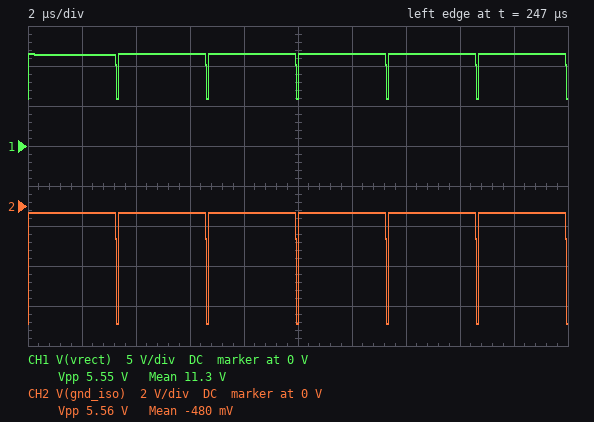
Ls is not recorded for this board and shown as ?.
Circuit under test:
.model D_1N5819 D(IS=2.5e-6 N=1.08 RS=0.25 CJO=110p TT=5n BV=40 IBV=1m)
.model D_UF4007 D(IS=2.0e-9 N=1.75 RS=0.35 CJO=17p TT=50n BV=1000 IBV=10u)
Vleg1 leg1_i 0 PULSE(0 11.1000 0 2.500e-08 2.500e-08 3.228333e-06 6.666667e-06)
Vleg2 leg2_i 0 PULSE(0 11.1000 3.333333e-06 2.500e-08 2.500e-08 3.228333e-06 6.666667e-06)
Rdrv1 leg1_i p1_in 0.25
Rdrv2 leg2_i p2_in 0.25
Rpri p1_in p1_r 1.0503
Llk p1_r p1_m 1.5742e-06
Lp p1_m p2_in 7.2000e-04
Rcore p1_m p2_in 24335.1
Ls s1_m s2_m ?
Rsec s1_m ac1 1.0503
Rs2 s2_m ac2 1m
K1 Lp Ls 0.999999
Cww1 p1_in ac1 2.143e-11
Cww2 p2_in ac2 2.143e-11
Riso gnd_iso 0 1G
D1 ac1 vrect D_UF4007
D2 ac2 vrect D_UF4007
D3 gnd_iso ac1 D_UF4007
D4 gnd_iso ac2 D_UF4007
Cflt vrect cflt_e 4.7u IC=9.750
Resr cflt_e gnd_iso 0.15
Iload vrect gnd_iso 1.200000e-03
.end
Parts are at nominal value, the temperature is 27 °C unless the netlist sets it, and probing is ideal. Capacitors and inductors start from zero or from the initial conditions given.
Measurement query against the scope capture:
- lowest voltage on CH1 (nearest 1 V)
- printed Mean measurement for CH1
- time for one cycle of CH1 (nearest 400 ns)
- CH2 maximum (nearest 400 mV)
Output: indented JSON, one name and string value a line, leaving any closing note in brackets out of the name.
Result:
{
  "lowest voltage on CH1": "6 V",
  "printed Mean measurement for CH1": "11.3 V",
  "time for one cycle of CH1": "3.2 µs",
  "CH2 maximum": "-400 mV"
}
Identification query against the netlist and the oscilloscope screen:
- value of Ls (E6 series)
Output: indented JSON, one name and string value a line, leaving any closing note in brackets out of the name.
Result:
{
  "value of Ls": "1 mH"
}
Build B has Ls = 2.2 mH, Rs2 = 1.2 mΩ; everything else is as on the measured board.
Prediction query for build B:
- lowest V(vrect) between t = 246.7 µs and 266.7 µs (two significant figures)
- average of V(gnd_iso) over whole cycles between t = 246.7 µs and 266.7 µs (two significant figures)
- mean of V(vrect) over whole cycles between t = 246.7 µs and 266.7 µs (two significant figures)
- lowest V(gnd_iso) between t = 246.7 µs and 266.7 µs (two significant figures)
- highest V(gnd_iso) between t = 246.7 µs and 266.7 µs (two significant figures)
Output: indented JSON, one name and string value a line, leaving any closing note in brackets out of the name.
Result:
{
  "lowest V(vrect) between t = 246.7 µs and 266.7 µs": "9.0 V",
  "average of V(gnd_iso) over whole cycles between t = 246.7 µs and 266.7 µs": "-3.6 V",
  "mean of V(vrect) over whole cycles between t = 246.7 µs and 266.7 µs": "14 V",
  "lowest V(gnd_iso) between t = 246.7 µs and 266.7 µs": "-9.0 V",
  "highest V(gnd_iso) between t = 246.7 µs and 266.7 µs": "-3.4 V"
}
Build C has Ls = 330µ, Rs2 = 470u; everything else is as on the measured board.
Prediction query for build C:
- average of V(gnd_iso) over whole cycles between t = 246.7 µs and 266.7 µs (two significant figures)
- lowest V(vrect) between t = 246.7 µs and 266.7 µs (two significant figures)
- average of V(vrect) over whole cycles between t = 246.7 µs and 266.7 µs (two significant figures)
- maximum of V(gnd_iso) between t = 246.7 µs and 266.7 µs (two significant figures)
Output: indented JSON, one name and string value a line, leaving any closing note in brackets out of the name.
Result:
{
  "average of V(gnd_iso) over whole cycles between t = 246.7 µs and 266.7 µs": "570 mV",
  "lowest V(vrect) between t = 246.7 µs and 266.7 µs": "4.8 V",
  "average of V(vrect) over whole cycles between t = 246.7 µs and 266.7 µs": "10 V",
  "maximum of V(gnd_iso) between t = 246.7 µs and 266.7 µs": "700 mV"
}
